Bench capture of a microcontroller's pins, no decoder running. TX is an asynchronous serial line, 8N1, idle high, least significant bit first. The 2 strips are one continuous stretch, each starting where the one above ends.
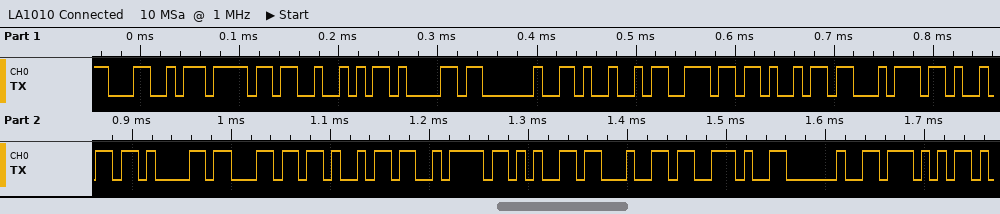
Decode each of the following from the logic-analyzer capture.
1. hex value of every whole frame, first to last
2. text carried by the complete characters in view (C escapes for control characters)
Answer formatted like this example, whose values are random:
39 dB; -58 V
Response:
4C 6F 52 61 20 49 6E 69 74 69 61 6C 69 7A 65 64 2E 20 57; "LoRa Initialized. W"
